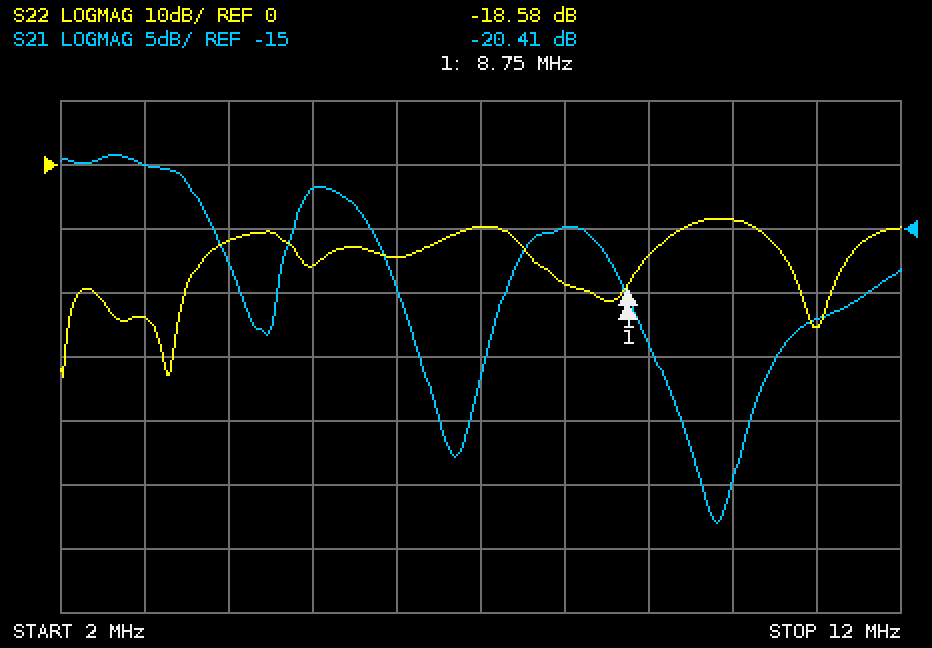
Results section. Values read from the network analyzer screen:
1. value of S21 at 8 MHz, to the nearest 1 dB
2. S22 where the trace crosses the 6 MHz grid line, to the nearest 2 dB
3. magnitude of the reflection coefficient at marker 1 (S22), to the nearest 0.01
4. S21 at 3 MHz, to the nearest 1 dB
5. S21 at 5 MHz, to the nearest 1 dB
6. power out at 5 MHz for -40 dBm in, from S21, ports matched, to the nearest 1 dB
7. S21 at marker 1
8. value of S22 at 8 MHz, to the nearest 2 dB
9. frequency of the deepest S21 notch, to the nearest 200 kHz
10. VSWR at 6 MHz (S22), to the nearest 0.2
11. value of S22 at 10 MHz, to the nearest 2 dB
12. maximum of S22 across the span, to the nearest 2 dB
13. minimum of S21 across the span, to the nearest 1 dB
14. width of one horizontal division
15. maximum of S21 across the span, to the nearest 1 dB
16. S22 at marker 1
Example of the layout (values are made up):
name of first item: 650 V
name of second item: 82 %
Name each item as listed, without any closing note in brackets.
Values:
value of S21 at 8 MHz, to the nearest 1 dB: -15 dB
S22 where the trace crosses the 6 MHz grid line, to the nearest 2 dB: -14 dB
magnitude of the reflection coefficient at marker 1 (S22), to the nearest 0.01: 0.12
S21 at 3 MHz, to the nearest 1 dB: -10 dB
S21 at 5 MHz, to the nearest 1 dB: -12 dB
power out at 5 MHz for -40 dBm in, from S21, ports matched, to the nearest 1 dB: -52 dBm
S21 at marker 1: -20.41 dB
value of S22 at 8 MHz, to the nearest 2 dB: -18 dB
frequency of the deepest S21 notch, to the nearest 200 kHz: 9.8 MHz
VSWR at 6 MHz (S22), to the nearest 0.2: 1.4
value of S22 at 10 MHz, to the nearest 2 dB: -8 dB
maximum of S22 across the span, to the nearest 2 dB: -8 dB
minimum of S21 across the span, to the nearest 1 dB: -38 dB
width of one horizontal division: 1 MHz
maximum of S21 across the span, to the nearest 1 dB: -9 dB
S22 at marker 1: -18.58 dB
